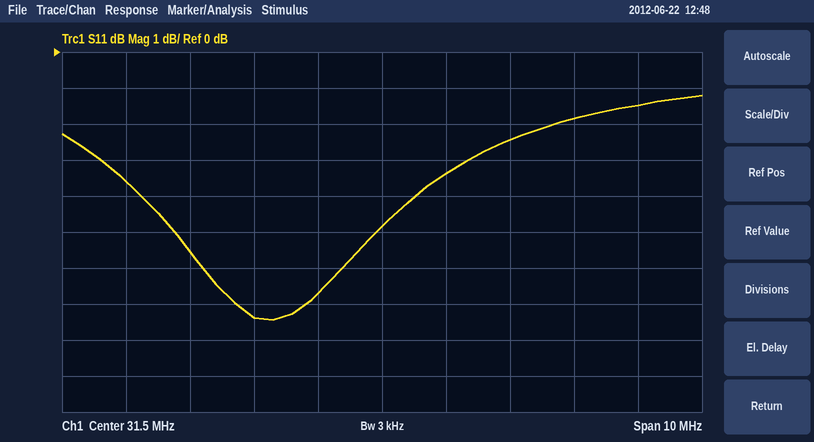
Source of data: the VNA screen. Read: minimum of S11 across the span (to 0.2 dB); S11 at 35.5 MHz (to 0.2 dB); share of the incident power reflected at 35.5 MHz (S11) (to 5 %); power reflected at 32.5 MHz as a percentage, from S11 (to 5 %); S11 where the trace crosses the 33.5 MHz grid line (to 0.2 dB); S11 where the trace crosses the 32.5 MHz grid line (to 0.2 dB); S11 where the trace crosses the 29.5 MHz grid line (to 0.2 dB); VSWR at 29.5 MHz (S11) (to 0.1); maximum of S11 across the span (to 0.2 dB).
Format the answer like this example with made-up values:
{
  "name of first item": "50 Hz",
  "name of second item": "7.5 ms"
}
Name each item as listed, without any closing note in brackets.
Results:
{
  "minimum of S11 across the span": "-7.4 dB",
  "S11 at 35.5 MHz": "-1.4 dB",
  "share of the incident power reflected at 35.5 MHz (S11)": "70 %",
  "power reflected at 32.5 MHz as a percentage, from S11": "45 %",
  "S11 where the trace crosses the 33.5 MHz grid line": "-2.4 dB",
  "S11 where the trace crosses the 32.5 MHz grid line": "-3.4 dB",
  "S11 where the trace crosses the 29.5 MHz grid line": "-7.4 dB",
  "VSWR at 29.5 MHz (S11)": "2.5",
  "maximum of S11 across the span": "-1.2 dB"
}
